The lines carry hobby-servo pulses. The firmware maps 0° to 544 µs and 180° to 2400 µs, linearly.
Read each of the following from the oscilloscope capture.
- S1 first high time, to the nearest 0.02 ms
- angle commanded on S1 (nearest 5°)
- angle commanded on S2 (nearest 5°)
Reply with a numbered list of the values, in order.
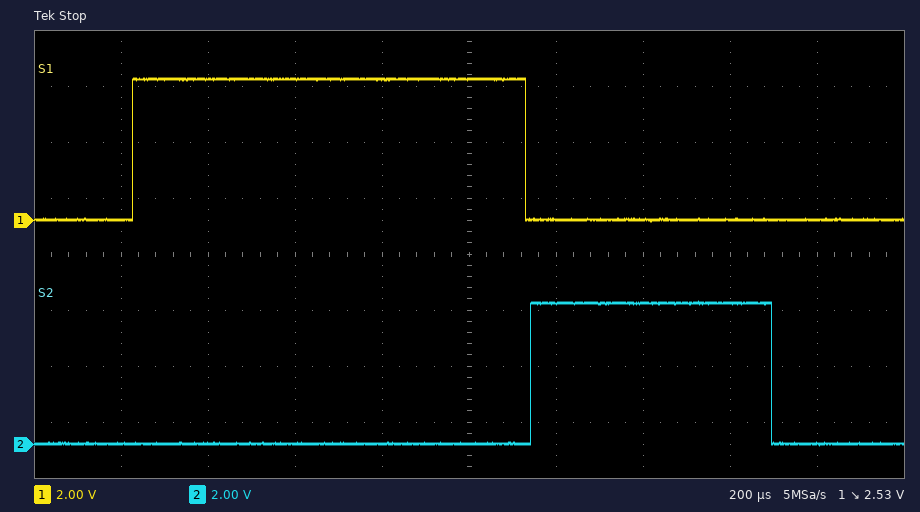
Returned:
1. 0.90 ms
2. 35°
3. 0°
